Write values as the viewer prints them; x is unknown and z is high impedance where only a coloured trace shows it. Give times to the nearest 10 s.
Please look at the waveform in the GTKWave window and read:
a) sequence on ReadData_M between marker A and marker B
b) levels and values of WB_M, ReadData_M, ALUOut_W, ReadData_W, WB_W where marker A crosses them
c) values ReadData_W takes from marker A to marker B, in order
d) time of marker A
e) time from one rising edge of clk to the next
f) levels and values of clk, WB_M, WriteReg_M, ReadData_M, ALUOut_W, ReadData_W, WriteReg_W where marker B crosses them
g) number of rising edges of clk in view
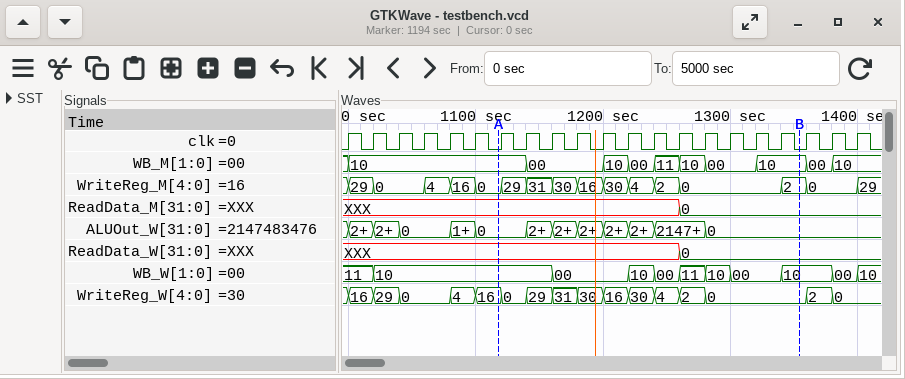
XXX, 0
WB_M=10, ReadData_M=XXX, ALUOut_W=0, ReadData_W=XXX, WB_W=10
XXX, 0
1120 s
20 s
clk=0, WB_M=10, WriteReg_M=2, ReadData_M=0, ALUOut_W=0, ReadData_W=0, WriteReg_W=0
21
